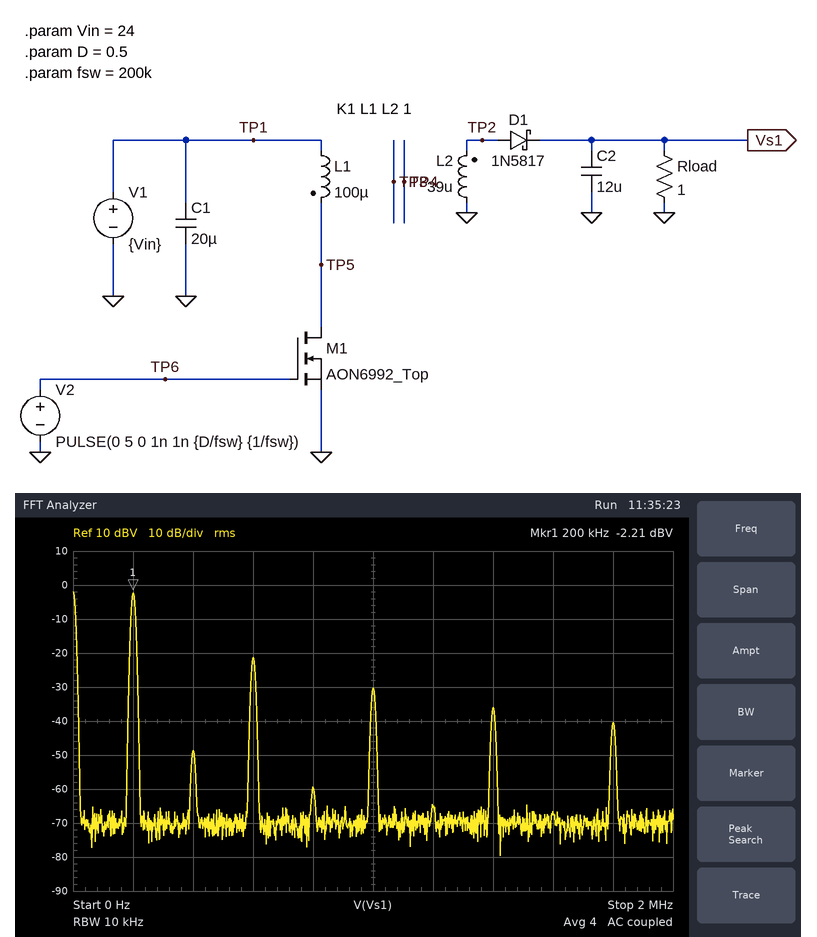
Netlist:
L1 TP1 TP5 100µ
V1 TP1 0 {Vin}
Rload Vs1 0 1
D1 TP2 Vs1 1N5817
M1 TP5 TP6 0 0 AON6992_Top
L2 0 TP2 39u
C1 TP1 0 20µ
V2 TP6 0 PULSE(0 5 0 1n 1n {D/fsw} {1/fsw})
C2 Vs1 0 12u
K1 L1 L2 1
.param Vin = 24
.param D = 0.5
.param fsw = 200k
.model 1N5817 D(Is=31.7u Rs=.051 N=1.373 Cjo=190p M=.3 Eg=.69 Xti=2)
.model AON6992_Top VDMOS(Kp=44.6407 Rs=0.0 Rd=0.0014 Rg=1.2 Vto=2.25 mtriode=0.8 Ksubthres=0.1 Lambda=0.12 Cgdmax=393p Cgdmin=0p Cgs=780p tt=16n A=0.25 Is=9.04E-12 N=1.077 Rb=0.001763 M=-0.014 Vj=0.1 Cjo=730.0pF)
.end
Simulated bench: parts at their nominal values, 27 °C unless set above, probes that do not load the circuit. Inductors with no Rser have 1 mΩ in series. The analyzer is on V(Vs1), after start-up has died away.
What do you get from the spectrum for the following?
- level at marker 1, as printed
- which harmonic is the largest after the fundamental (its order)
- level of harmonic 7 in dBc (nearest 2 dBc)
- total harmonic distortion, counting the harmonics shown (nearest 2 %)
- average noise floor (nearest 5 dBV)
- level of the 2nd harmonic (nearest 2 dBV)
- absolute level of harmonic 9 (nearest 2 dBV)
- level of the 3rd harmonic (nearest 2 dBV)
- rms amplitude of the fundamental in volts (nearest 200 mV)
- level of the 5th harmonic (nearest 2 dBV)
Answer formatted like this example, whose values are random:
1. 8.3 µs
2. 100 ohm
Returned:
1. -2.21 dBV
2. 3
3. -34 dBc
4. 12 %
5. -70 dBV
6. -48 dBV
7. -40 dBV
8. -22 dBV
9. 800 mV
10. -30 dBV
